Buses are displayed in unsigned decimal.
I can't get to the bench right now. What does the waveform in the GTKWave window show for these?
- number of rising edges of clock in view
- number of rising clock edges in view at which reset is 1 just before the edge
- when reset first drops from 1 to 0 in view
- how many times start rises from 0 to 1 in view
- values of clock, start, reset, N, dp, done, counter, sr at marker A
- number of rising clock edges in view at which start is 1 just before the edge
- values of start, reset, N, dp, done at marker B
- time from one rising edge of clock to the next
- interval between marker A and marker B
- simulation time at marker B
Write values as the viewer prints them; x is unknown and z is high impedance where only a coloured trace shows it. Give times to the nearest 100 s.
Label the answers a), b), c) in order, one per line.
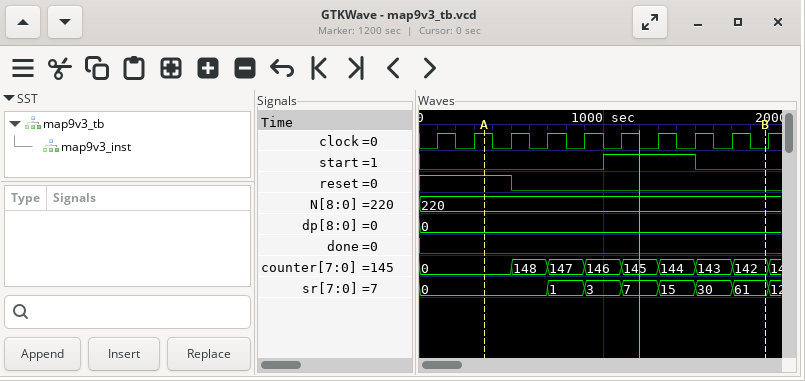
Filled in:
a) 10
b) 3
c) 500 s
d) 1
e) clock=1, start=0, reset=1, N=220, dp=0, done=0, counter=0, sr=0
f) 3
g) start=0, reset=0, N=220, dp=0, done=0
h) 200 s
i) 1500 s
j) 1900 s
